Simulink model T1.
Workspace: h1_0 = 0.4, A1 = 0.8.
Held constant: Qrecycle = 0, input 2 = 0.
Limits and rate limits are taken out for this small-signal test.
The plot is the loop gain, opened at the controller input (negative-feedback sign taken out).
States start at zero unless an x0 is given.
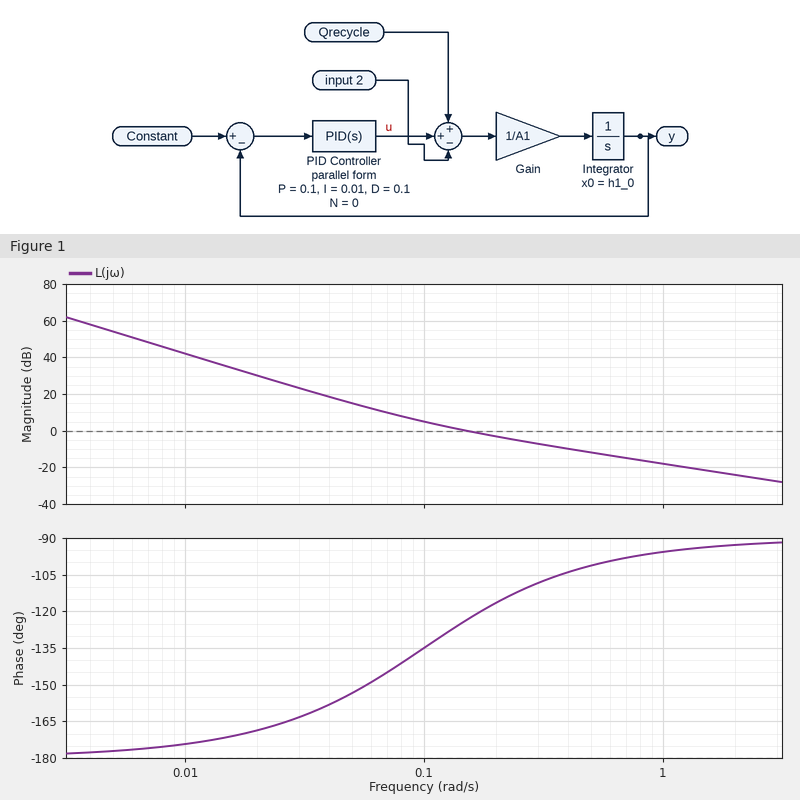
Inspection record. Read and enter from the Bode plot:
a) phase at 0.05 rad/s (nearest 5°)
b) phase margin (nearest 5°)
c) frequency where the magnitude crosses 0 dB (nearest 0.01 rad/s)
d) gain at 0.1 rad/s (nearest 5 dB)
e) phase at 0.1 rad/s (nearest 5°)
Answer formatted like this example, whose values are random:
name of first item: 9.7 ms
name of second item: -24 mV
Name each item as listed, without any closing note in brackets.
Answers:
phase at 0.05 rad/s: -155°
phase margin: 55°
frequency where the magnitude crosses 0 dB: 0.15 rad/s
gain at 0.1 rad/s: 5 dB
phase at 0.1 rad/s: -135°
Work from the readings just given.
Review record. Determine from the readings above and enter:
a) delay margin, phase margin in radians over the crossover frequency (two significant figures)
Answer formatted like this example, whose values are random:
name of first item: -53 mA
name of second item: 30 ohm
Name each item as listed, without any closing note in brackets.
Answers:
delay margin, phase margin in radians over the crossover frequency: 6.4 s
